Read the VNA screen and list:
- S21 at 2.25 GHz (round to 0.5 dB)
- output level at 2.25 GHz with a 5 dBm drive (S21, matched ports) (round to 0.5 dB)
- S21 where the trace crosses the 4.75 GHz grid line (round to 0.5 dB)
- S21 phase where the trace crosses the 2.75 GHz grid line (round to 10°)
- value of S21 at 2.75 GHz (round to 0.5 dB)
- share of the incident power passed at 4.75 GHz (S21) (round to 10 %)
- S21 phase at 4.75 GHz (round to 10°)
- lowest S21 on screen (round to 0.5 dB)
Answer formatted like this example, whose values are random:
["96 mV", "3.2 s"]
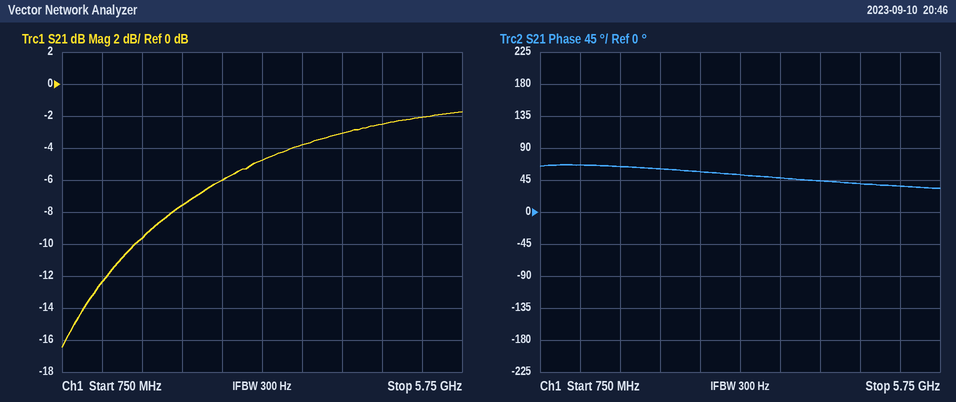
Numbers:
["-7.5 dB", "-2.5 dBm", "-2.5 dB", "60°", "-6.0 dB", "60 %", "40°", "-16.5 dB"]
